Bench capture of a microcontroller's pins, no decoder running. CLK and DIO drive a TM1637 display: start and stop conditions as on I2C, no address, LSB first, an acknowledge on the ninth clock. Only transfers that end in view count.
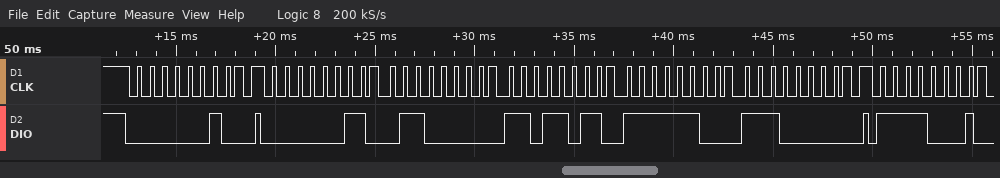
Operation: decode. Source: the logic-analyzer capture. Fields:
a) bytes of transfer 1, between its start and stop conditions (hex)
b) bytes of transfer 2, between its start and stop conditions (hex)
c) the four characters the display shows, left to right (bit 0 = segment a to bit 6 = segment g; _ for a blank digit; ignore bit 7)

40
C0 06 DB 3F 07
1207
